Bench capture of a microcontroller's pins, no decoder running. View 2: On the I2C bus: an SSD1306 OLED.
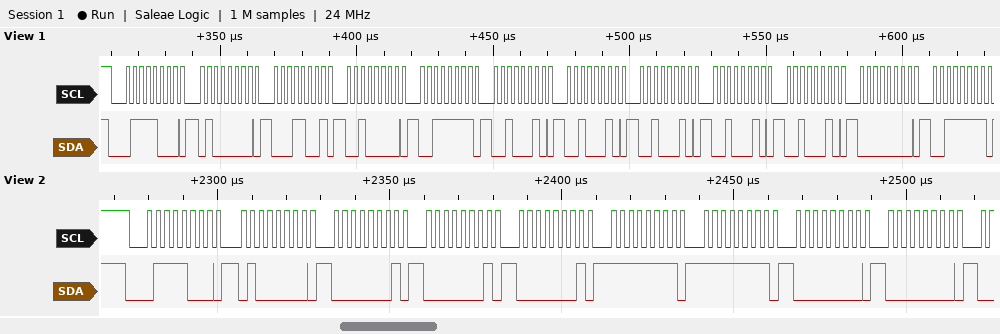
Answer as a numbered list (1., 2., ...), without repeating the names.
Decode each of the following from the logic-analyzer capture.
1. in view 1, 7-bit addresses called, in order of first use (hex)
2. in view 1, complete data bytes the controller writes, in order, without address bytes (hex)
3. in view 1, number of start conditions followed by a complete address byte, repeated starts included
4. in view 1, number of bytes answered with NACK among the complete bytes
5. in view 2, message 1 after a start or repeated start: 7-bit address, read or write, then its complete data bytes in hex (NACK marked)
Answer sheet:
1. 0x3C
2. 40 19 20 3F 22 22 22 22 22 00 3F
3. 1
4. 0
5. 0x3C write: 40 01 01 01 FF FF 00 00
